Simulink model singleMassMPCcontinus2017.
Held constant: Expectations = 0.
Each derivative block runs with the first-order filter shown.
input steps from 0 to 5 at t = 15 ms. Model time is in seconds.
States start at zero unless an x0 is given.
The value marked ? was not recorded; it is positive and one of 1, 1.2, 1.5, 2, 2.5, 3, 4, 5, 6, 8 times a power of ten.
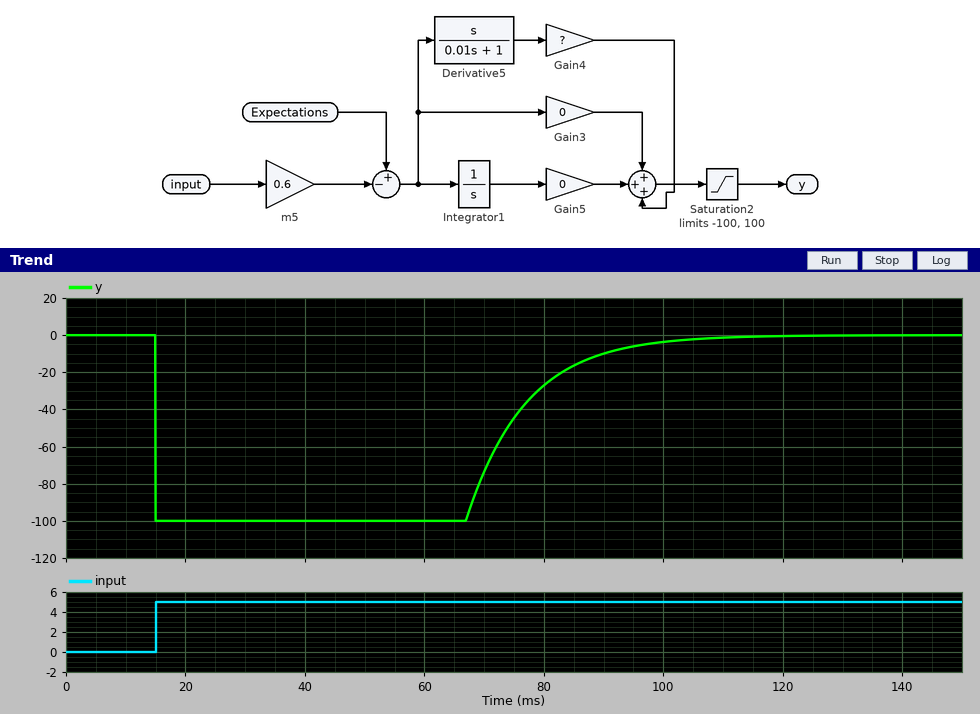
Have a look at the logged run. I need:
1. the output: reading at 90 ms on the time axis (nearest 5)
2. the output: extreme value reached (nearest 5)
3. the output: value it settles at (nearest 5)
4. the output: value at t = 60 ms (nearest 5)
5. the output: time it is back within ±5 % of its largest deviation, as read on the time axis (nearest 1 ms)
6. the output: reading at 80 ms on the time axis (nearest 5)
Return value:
-10
-100
0
-100
97 ms
-25
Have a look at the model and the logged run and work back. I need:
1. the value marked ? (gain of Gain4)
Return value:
60
